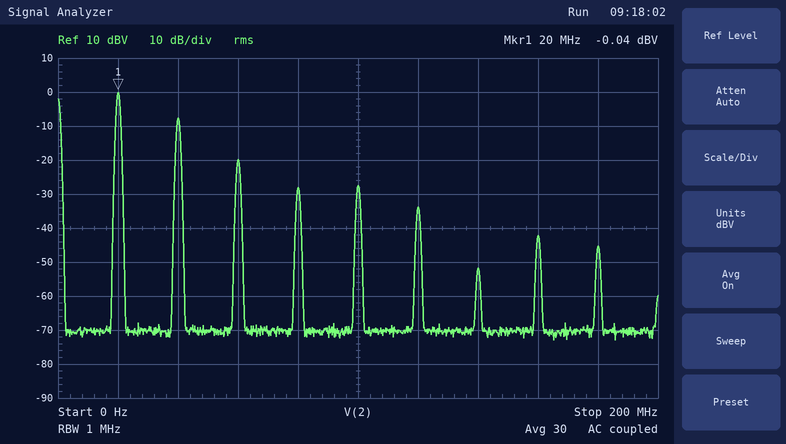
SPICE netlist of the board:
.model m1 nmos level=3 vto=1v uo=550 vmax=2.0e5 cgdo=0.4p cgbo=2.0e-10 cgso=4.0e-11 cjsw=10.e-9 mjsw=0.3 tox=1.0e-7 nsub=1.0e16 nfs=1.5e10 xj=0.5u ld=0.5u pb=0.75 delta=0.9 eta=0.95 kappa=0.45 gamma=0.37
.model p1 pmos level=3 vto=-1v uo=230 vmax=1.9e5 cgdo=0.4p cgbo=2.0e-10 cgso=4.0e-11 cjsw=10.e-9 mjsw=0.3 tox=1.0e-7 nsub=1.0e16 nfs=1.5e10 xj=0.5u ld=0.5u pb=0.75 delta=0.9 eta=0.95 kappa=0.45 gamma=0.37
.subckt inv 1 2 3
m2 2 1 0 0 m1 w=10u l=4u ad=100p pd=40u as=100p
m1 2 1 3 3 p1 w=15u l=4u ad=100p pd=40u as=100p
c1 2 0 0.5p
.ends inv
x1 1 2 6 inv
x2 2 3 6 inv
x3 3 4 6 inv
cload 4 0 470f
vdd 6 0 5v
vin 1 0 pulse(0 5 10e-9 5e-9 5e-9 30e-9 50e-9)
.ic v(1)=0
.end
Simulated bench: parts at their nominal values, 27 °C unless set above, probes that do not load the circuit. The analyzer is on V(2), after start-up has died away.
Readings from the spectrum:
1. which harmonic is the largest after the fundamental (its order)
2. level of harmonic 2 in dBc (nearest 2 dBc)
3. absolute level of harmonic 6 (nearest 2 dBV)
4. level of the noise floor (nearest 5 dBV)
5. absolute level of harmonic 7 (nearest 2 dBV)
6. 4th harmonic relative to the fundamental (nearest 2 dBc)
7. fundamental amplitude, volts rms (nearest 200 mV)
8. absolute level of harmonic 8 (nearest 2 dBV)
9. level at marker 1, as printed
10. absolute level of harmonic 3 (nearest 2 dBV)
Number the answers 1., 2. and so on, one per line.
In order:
1. 2
2. -8 dBc
3. -34 dBV
4. -70 dBV
5. -52 dBV
6. -28 dBc
7. 1.0 V
8. -42 dBV
9. -0.04 dBV
10. -20 dBV
